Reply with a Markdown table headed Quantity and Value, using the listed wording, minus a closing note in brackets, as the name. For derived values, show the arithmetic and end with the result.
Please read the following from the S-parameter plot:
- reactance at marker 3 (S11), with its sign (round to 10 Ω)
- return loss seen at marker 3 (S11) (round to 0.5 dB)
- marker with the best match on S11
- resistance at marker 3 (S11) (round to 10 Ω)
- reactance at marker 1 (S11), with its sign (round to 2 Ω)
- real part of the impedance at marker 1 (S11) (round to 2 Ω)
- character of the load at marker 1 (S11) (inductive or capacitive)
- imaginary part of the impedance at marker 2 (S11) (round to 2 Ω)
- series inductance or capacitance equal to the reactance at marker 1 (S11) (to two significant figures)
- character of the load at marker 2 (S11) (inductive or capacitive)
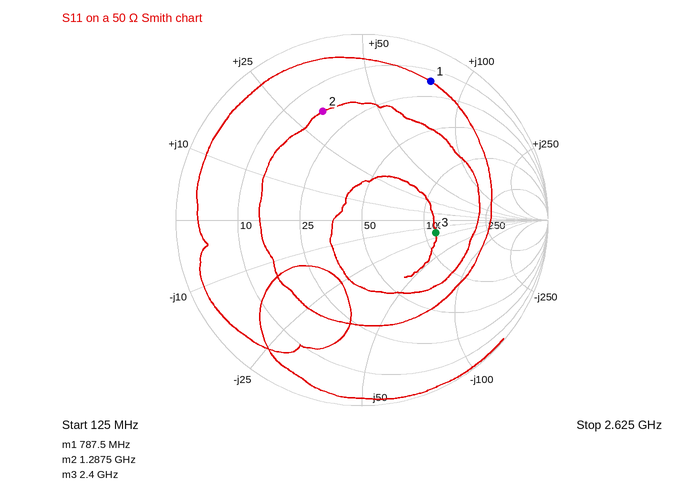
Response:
| Quantity | Value |
|---|---|
| reactance at marker 3 (S11), with its sign | -20 Ω |
| return loss seen at marker 3 (S11) | 8.0 dB |
| marker with the best match on S11 | marker 3 |
| resistance at marker 3 (S11) | 110 Ω |
| reactance at marker 1 (S11), with its sign | +78 Ω |
| real part of the impedance at marker 1 (S11) | 16 Ω |
| character of the load at marker 1 (S11) | inductive |
| imaginary part of the impedance at marker 2 (S11) | +32 Ω |
| series inductance or capacitance equal to the reactance at marker 1 (S11) | L = 78 Ω/(2π × 787.5 MHz) ≈ 16 nH |
| character of the load at marker 2 (S11) | inductive |
